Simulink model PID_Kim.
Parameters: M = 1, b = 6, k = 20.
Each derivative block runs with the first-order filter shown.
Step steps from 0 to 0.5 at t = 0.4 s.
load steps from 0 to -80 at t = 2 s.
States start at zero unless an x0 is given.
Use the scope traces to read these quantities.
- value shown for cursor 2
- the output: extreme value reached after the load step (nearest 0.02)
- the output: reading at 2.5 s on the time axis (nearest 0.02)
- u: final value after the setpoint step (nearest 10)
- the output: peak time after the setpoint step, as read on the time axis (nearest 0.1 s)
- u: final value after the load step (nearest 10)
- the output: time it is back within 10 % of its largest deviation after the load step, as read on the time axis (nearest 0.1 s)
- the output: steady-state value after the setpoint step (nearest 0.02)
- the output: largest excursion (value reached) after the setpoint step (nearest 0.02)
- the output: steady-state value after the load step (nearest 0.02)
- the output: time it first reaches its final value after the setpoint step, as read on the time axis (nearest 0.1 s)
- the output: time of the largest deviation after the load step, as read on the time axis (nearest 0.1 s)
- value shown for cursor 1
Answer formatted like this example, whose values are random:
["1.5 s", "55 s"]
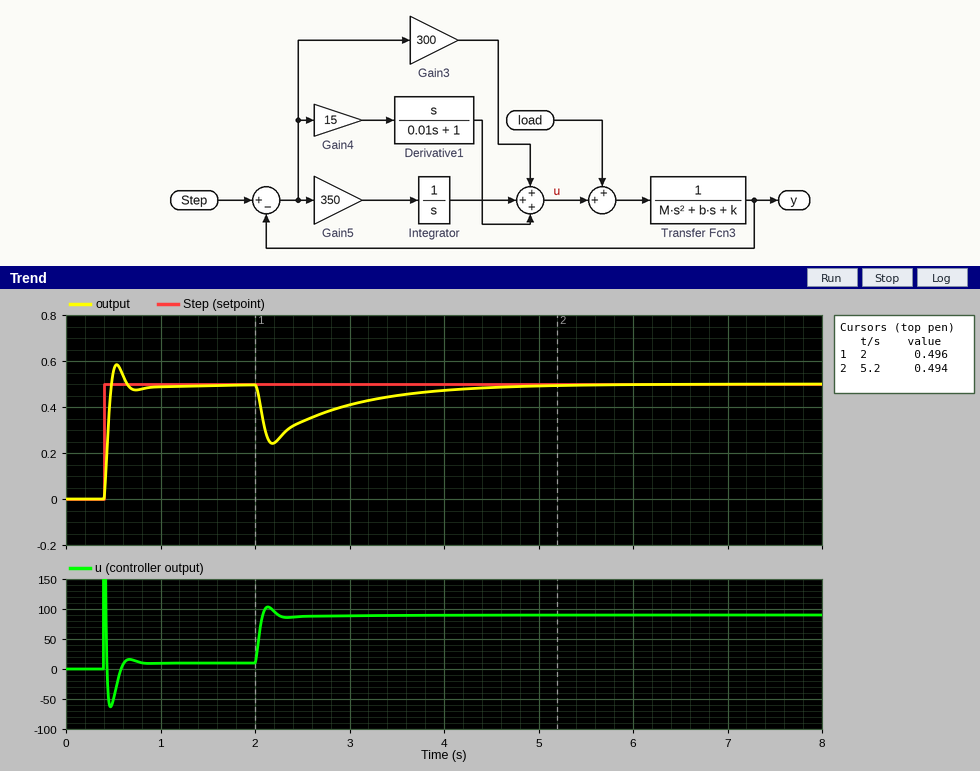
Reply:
["0.494", "0.24", "0.34", "10", "0.5 s", "90", "4.1 s", "0.50", "0.58", "0.50", "0.5 s", "2.2 s", "0.496"]
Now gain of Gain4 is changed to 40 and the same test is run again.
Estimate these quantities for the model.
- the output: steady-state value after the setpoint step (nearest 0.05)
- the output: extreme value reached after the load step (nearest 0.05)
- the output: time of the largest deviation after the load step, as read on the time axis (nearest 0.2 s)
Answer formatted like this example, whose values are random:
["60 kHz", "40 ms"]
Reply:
["0.50", "0.30", "2.4 s"]
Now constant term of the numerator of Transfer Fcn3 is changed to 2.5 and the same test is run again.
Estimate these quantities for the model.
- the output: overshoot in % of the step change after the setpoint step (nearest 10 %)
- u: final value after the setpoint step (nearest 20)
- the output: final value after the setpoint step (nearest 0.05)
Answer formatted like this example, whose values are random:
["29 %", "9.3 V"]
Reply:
["20 %", "0", "0.50"]
